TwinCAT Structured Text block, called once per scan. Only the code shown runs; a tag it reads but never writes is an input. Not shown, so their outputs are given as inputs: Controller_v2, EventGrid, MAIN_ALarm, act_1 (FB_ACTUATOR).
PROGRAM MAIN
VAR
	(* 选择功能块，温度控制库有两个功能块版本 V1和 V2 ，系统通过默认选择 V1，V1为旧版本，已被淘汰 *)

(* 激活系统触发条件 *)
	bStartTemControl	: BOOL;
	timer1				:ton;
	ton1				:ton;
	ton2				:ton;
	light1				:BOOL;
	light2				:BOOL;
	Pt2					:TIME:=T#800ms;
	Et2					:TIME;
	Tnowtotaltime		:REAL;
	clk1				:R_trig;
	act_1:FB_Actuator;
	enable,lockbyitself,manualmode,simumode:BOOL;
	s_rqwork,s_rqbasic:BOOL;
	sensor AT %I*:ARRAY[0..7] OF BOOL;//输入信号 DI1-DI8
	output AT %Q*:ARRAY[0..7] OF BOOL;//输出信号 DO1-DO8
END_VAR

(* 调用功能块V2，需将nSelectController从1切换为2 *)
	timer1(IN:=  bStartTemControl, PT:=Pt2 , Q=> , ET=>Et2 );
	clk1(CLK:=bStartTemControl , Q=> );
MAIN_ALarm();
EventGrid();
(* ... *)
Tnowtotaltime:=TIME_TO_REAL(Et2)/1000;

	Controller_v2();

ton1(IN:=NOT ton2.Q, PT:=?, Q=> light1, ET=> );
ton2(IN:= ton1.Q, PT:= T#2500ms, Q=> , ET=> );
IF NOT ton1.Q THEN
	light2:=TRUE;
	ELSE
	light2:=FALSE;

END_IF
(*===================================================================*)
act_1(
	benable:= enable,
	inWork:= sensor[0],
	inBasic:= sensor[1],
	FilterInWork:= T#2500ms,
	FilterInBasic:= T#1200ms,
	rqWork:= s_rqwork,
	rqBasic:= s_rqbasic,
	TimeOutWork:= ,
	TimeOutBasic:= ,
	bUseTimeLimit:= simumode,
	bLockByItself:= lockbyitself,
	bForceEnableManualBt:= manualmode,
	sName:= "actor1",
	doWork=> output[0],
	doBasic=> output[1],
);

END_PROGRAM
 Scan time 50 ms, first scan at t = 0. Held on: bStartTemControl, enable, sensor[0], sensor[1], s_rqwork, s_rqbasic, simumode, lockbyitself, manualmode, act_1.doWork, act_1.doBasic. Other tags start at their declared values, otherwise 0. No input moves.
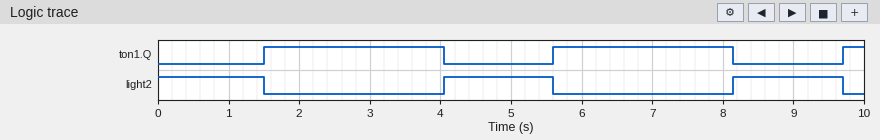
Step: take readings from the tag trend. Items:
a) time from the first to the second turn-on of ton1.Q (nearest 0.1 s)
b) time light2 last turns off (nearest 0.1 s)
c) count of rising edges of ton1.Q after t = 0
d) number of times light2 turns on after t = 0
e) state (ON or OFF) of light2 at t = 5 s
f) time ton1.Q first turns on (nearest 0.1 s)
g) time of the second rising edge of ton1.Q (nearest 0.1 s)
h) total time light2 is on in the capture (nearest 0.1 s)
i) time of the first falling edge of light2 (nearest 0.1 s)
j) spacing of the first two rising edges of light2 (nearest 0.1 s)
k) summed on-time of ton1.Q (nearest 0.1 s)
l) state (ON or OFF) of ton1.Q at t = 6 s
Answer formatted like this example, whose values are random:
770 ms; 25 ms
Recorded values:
4.1 s; 9.7 s; 3; 2; ON; 1.5 s; 5.6 s; 4.6 s; 1.5 s; 4.1 s; 5.4 s; ON
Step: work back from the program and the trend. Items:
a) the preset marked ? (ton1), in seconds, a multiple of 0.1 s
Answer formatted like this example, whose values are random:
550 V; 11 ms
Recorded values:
1.5 s
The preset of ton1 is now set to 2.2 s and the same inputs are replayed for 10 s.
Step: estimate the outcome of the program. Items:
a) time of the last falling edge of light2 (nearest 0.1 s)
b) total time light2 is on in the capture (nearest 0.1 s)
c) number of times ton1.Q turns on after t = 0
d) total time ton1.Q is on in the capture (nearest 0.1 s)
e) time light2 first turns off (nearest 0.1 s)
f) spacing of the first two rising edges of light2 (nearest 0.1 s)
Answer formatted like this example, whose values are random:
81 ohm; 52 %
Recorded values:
7.0 s; 4.9 s; 2; 5.1 s; 2.2 s; 4.8 s
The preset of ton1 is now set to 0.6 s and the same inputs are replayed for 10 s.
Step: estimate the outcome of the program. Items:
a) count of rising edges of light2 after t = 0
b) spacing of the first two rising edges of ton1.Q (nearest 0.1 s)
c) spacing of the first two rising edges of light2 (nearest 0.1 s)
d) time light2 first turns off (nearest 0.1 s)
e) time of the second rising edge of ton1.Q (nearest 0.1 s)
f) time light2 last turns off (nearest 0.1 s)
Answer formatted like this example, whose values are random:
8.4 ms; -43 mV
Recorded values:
3; 3.2 s; 3.2 s; 0.6 s; 3.8 s; 7.0 s
